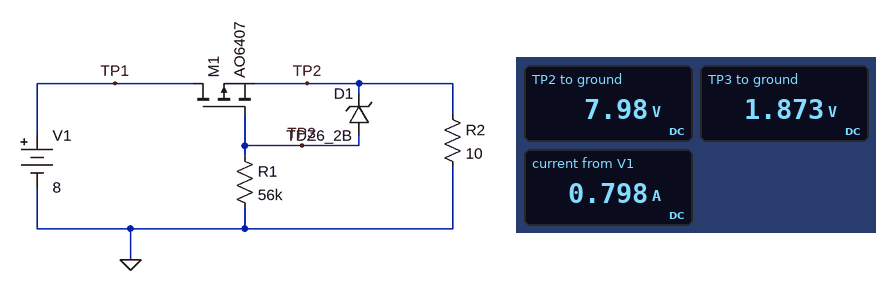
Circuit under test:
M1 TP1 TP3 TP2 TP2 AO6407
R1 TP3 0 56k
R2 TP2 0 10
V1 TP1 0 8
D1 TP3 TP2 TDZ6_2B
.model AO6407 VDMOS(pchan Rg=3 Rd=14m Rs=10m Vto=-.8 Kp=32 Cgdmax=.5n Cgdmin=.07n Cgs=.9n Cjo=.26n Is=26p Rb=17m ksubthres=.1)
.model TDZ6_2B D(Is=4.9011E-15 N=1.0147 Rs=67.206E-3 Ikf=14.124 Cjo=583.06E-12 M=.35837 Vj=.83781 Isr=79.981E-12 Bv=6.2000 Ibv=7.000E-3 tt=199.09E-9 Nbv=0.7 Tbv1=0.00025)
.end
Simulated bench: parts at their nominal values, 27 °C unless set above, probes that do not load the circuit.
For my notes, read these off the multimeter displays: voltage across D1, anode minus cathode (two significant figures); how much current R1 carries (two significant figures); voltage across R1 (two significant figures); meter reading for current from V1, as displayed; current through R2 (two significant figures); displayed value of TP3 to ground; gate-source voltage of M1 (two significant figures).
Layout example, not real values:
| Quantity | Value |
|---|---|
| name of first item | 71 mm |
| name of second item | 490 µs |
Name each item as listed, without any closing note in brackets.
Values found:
| Quantity | Value |
|---|---|
| voltage across D1, anode minus cathode | -6.1 V |
| how much current R1 carries | 33 µA |
| voltage across R1 | 1.9 V |
| meter reading for current from V1, as displayed | 0.798 A |
| current through R2 | 800 mA |
| displayed value of TP3 to ground | 1.873 V |
| gate-source voltage of M1 | -6.1 V |
